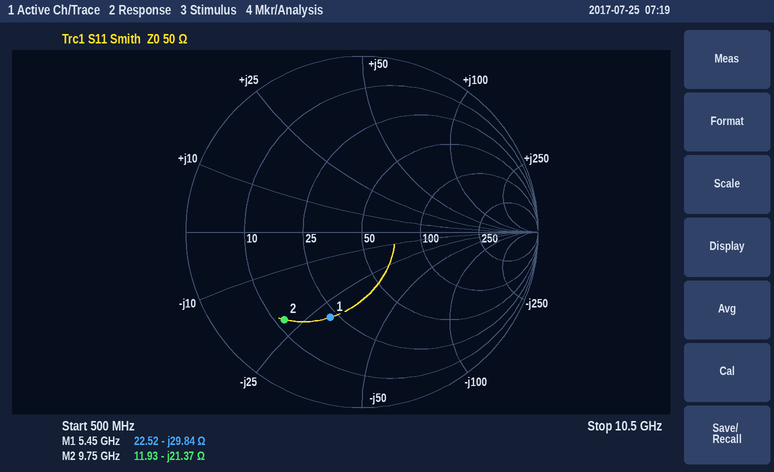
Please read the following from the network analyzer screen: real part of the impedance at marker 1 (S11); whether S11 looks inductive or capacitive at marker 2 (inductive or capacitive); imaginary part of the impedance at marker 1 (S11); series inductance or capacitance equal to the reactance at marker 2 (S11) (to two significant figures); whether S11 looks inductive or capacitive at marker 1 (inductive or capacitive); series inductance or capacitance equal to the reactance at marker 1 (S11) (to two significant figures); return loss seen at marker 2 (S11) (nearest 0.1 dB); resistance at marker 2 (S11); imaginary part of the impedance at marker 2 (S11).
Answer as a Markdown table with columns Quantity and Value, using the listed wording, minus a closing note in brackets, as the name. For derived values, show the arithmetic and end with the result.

| Quantity | Value |
|---|---|
| real part of the impedance at marker 1 | 22.52 Ω |
| whether S11 looks inductive or capacitive at marker 2 | capacitive |
| imaginary part of the impedance at marker 1 | -29.84 Ω |
| series inductance or capacitance equal to the reactance at marker 2 (S11) | C = 1/(2π × 9.75 GHz × 21.37 Ω) ≈ 764 fF, so 760 fF to two significant figures |
| whether S11 looks inductive or capacitive at marker 1 | capacitive |
| series inductance or capacitance equal to the reactance at marker 1 (S11) | C = 1/(2π × 5.45 GHz × 29.84 Ω) ≈ 979 fF, so 980 fF to two significant figures |
| return loss seen at marker 2 (S11) | 3.5 dB |
| resistance at marker 2 | 11.93 Ω |
| imaginary part of the impedance at marker 2 | -21.37 Ω |
